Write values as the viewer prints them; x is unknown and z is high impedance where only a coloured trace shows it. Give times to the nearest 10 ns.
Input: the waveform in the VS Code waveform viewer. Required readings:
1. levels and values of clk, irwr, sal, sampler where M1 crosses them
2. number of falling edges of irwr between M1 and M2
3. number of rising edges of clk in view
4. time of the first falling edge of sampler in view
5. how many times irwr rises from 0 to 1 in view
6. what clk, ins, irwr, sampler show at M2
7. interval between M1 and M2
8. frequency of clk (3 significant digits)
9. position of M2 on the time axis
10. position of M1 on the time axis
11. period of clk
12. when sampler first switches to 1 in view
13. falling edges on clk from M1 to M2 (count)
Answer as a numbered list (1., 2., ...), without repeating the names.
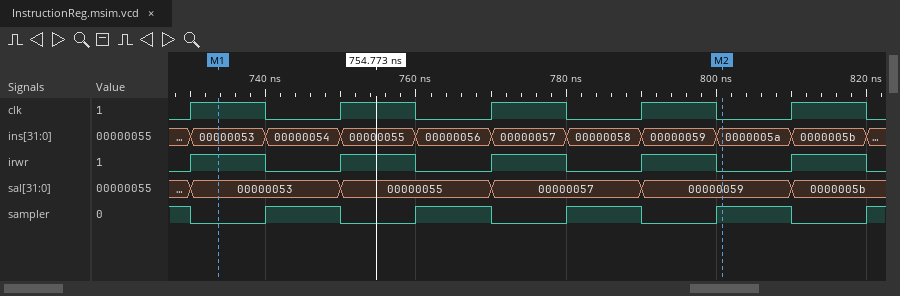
1. clk=1, irwr=1, sal=00000053, sampler=0
2. 4
3. 5
4. 730 ns
5. 5
6. clk=0, ins=0000005a, irwr=0, sampler=1
7. 70 ns
8. 50.0 MHz
9. 800 ns
10. 730 ns
11. 20 ns
12. 740 ns
13. 4
